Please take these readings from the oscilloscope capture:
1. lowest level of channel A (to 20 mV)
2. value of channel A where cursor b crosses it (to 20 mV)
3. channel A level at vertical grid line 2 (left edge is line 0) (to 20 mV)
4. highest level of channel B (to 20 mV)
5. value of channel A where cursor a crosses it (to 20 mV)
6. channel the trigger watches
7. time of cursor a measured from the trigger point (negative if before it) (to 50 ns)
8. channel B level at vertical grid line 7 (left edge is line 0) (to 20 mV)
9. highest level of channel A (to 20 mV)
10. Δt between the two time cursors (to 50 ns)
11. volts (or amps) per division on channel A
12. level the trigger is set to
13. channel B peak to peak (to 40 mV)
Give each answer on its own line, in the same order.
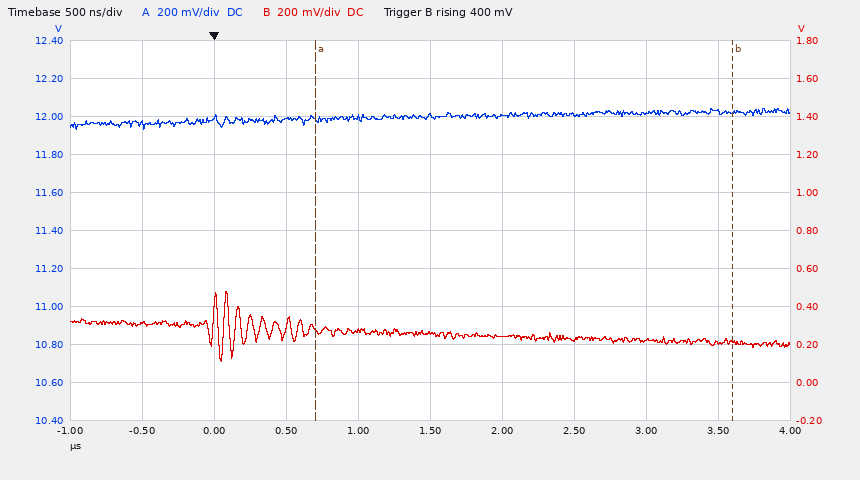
11.94 V
12.02 V
12.00 V
480 mV
11.98 V
channel B
+700 ns
220 mV
12.04 V
2.90 µs
200 mV
400 mV
360 mV
